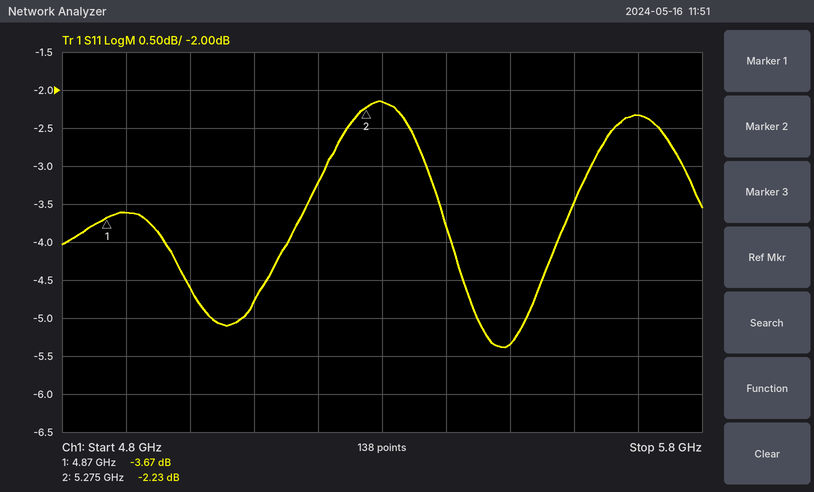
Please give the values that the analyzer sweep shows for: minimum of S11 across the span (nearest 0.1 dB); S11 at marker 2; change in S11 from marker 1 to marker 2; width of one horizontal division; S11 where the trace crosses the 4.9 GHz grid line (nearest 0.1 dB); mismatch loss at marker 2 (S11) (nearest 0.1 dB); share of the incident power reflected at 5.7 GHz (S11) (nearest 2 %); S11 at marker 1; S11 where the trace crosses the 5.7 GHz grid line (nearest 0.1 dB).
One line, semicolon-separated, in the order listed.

-5.4 dB; -2.23 dB; 1.44 dB; 100 MHz; -3.6 dB; 4.0 dB; 58 %; -3.67 dB; -2.3 dB
